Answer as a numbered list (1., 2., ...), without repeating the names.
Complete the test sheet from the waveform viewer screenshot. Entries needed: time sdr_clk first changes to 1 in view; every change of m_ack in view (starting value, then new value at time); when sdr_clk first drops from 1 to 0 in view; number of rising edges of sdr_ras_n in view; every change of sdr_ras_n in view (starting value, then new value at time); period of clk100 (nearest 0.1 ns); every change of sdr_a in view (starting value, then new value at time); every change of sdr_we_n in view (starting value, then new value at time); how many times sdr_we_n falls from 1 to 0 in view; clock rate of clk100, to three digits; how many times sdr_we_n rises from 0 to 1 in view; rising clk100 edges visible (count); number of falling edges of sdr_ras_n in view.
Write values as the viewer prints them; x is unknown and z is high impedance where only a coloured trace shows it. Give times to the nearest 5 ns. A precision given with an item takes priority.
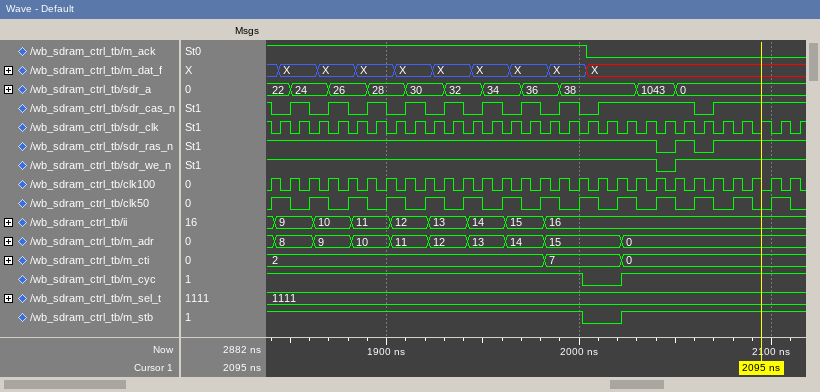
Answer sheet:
1. 1845 ns
2. 1, 0 at 2005 ns
3. 1840 ns
4. 2
5. 1, 0 at 2040 ns, 1 at 2050 ns, 0 at 2060 ns, 1 at 2070 ns
6. 10 ns
7. 22, 24 at 1850 ns, 26 at 1870 ns, 28 at 1890 ns, 30 at 1910 ns, 32 at 1930 ns, 34 at 1950 ns, 36 at 1970 ns, 38 at 1990 ns, 1043 at 2030 ns, 0 at 2050 ns
8. 1, 0 at 2040 ns, 1 at 2050 ns
9. 1
10. 100 MHz
11. 1
12. 28
13. 2
